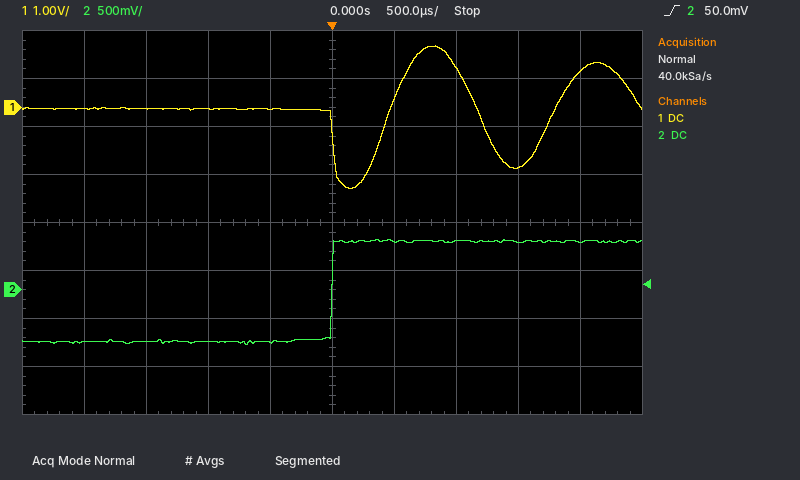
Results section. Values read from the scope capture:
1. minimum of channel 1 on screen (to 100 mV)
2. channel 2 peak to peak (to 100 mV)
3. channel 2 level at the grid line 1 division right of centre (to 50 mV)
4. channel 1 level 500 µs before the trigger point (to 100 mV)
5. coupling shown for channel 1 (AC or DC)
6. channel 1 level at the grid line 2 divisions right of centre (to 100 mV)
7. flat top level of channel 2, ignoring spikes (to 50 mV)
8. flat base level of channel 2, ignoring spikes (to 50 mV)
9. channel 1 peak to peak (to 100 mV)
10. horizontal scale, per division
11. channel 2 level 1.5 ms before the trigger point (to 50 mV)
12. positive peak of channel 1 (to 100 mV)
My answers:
-1.7 V
1.10 V
500 mV
0.0 V
DC
800 mV
500 mV
-550 mV
3.0 V
500 µs
-550 mV
1.3 V
